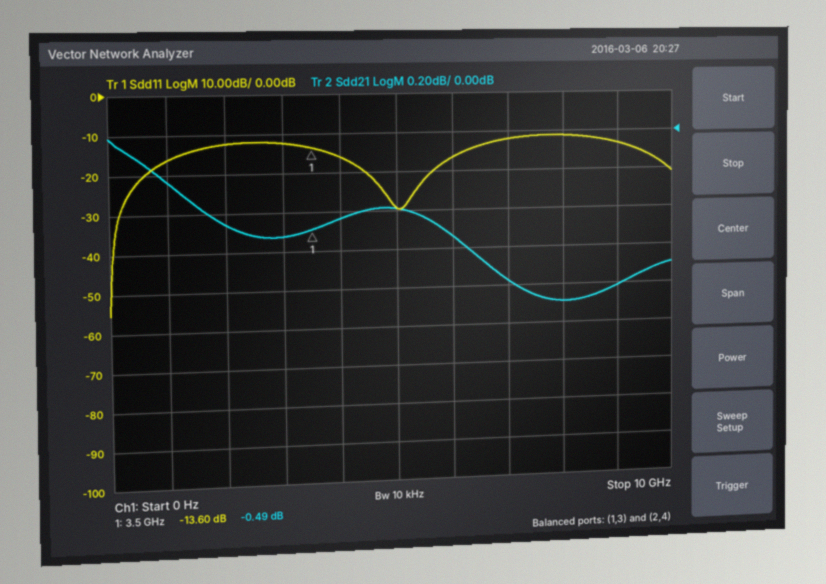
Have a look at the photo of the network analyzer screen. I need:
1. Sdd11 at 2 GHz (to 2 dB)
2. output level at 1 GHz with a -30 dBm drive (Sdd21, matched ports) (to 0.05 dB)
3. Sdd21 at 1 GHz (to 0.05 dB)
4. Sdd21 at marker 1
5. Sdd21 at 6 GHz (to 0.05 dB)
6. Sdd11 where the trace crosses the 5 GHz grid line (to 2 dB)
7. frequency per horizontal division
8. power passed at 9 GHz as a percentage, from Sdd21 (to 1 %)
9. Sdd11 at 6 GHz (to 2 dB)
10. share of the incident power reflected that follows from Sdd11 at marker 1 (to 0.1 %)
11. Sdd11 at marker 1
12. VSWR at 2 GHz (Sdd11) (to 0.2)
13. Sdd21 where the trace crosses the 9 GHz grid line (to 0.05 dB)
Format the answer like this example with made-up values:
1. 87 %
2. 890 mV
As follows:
1. -12 dB
2. -30.25 dBm
3. -0.25 dB
4. -0.49 dB
5. -0.55 dB
6. -30 dB
7. 1 GHz
8. 83 %
9. -16 dB
10. 4.4 %
11. -13.60 dB
12. 1.6
13. -0.80 dB
